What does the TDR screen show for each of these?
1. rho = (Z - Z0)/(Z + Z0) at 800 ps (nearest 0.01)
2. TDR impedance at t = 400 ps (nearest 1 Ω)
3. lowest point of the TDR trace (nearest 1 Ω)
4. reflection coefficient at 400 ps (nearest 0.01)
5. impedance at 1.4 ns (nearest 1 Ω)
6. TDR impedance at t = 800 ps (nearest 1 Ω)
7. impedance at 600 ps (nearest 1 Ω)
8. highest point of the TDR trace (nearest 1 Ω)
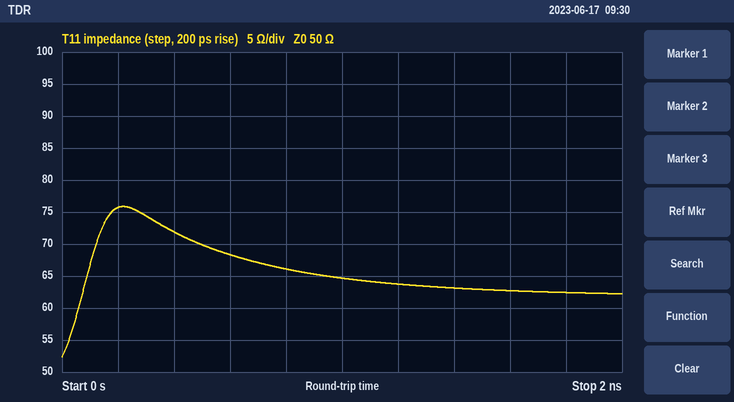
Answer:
+0.14
72 Ω
52 Ω
+0.18
63 Ω
66 Ω
68 Ω
76 Ω
